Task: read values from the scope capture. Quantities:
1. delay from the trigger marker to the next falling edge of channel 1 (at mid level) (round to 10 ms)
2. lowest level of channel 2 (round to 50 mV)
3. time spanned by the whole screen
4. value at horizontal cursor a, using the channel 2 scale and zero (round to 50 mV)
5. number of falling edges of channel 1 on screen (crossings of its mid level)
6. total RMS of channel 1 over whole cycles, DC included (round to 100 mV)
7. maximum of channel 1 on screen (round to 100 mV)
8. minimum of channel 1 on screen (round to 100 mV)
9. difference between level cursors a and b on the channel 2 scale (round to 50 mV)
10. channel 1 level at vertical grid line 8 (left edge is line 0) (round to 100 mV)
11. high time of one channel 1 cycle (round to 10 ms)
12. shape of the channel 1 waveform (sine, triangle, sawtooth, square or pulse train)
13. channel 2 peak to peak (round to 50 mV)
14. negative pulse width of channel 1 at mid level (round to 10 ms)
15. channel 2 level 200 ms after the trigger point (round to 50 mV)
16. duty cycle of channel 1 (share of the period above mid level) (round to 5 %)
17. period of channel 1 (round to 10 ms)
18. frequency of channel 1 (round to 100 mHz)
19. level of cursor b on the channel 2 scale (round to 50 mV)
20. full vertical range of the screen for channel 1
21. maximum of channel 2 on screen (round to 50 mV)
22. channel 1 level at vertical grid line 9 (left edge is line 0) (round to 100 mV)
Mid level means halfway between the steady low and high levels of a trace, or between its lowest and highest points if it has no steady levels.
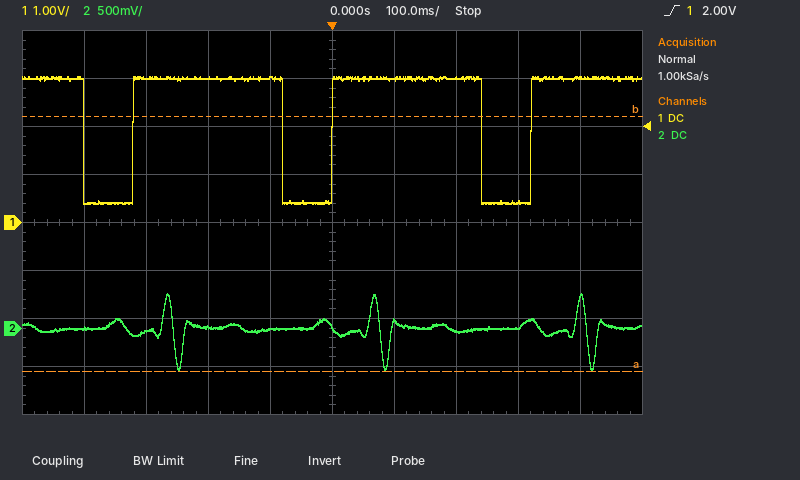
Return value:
240 ms
-450 mV
1 s
-450 mV
3
2.6 V
3.0 V
400 mV
2.65 V
400 mV
240 ms
pulse train
800 mV
80 ms
-50 mV
75 %
320 ms
3.1 Hz
2.20 V
8 V
350 mV
3.0 V
